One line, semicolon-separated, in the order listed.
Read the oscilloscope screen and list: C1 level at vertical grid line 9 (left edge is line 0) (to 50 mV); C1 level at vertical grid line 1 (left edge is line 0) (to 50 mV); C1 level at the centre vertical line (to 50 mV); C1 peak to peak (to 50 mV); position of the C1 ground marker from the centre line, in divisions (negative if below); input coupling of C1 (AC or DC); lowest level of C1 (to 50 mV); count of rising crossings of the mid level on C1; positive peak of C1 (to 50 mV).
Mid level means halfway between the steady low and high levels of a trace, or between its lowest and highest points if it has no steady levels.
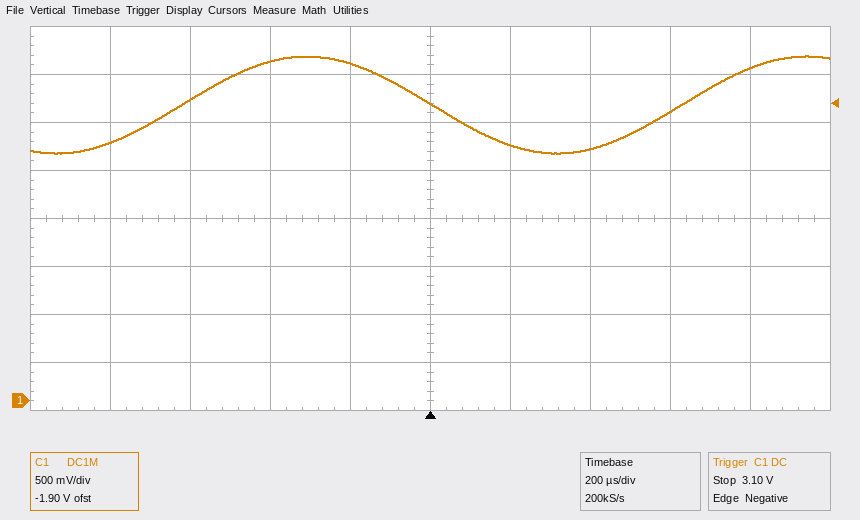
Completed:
3.45 V; 2.70 V; 3.10 V; 1.00 V; -3.8 div; DC; 2.60 V; 2; 3.60 V
